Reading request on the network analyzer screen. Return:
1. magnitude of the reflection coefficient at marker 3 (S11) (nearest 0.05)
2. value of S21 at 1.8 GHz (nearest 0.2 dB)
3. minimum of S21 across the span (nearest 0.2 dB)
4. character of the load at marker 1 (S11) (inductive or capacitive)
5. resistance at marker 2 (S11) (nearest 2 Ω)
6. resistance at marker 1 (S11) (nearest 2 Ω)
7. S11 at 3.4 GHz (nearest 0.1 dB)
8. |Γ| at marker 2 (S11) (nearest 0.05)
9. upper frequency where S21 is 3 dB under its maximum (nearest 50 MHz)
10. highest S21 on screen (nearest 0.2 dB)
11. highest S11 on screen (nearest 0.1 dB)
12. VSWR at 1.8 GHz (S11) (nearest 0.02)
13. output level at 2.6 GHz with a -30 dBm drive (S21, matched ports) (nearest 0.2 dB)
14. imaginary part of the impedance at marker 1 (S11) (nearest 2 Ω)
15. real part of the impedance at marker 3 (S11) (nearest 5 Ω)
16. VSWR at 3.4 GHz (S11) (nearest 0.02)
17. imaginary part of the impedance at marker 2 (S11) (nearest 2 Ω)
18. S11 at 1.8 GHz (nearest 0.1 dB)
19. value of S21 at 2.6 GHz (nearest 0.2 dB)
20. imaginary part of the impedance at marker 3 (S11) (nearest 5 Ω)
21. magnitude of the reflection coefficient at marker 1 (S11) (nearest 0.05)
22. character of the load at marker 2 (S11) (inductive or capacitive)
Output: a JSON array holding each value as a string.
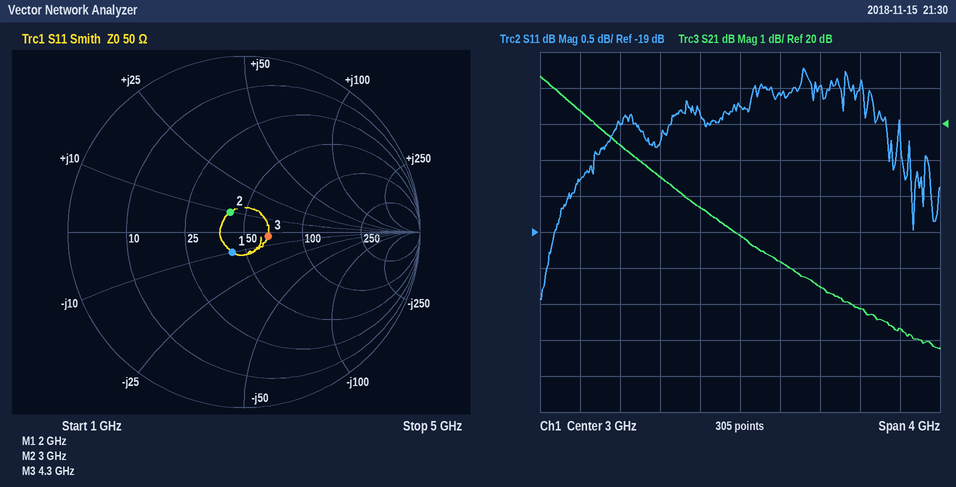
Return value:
["0.15", "19.4 dB", "13.8 dB", "capacitive", "42 Ω", "42 Ω", "-17.1 dB", "0.15", "2.30 GHz", "21.4 dB", "-16.7 dB", "1.30", "-12.4 dBm", "-10 Ω", "65 Ω", "1.32", "+10 Ω", "-17.5 dB", "17.6 dB", "-5 Ω", "0.15", "inductive"]
